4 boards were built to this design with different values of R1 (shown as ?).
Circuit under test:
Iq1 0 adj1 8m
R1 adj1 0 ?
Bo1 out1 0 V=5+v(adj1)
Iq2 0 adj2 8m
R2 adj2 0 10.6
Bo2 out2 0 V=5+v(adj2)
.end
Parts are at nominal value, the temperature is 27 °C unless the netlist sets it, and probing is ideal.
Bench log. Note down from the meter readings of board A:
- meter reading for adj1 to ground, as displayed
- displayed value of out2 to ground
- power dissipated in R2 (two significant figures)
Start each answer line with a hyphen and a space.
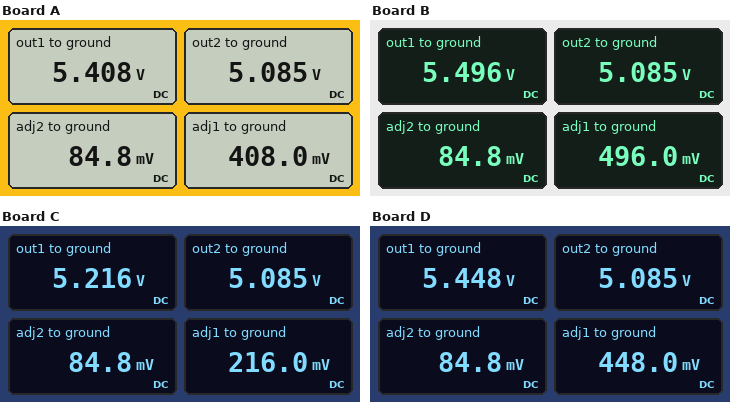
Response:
- 408.0 mV
- 5.085 V
- 680 µW
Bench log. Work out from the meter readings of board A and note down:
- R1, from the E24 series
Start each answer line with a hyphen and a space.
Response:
- 51 Ω
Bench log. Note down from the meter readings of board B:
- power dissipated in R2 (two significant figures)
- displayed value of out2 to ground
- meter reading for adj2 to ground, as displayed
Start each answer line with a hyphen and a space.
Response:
- 680 µW
- 5.085 V
- 84.8 mV
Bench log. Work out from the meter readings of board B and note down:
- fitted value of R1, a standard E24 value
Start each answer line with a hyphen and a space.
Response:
- 62 Ω
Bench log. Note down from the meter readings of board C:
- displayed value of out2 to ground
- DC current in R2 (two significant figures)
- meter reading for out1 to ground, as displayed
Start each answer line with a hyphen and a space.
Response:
- 5.085 V
- 8.0 mA
- 5.216 V
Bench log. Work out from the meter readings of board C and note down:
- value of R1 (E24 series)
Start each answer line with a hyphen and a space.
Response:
- 27 Ω
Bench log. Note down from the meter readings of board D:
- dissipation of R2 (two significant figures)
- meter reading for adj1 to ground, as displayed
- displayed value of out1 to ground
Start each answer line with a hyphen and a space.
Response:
- 680 µW
- 448.0 mV
- 5.448 V
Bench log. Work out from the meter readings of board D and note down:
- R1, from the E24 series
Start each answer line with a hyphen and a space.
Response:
- 56 Ω
